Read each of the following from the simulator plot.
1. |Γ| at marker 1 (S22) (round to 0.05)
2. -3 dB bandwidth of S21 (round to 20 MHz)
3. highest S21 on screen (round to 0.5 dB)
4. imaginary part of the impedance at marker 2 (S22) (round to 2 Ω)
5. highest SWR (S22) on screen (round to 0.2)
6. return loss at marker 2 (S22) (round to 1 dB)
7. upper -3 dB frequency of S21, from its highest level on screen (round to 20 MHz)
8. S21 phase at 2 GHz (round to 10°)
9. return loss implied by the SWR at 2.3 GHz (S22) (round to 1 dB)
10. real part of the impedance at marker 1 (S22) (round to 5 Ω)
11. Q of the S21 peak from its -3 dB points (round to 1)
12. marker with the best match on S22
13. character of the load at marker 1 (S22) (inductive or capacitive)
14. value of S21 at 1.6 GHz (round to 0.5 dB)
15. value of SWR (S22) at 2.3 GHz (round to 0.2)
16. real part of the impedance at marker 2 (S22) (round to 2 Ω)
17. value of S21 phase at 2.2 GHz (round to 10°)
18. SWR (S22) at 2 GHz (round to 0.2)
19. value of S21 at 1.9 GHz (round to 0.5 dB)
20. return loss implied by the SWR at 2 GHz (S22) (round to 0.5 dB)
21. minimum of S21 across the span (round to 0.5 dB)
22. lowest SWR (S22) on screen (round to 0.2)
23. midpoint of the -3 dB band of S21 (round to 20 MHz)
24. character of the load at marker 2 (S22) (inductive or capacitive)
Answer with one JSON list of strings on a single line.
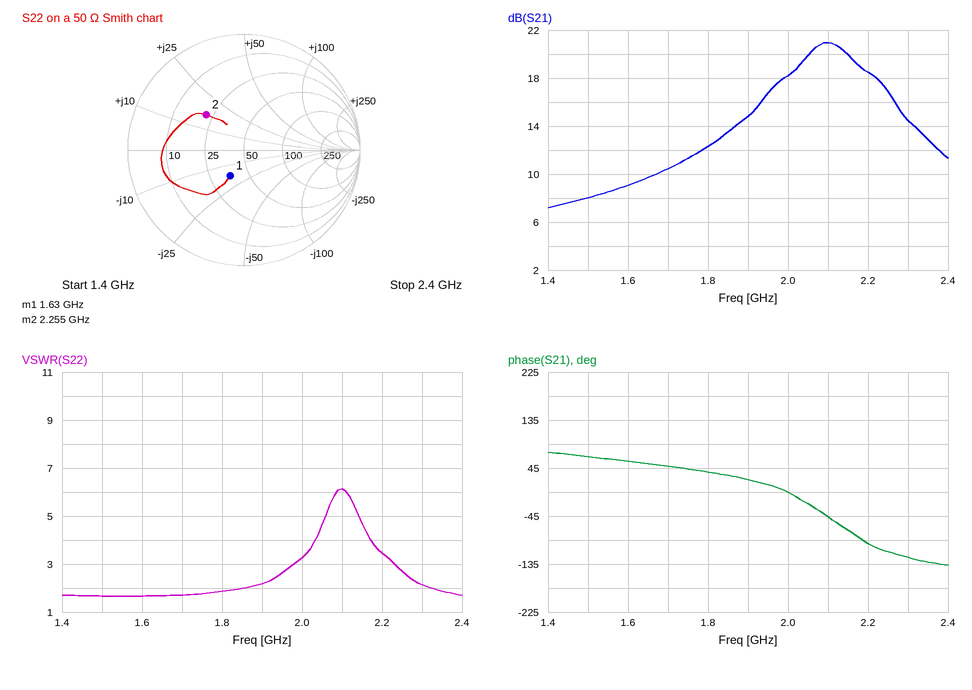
["0.25", "240 MHz", "21.0 dB", "+16 Ω", "6.2", "7 dB", "2.22 GHz", "0°", "9 dB", "35 Ω", "9", "marker 1", "capacitive", "9.0 dB", "2.2", "22 Ω", "-100°", "3.2", "15.0 dB", "5.5 dB", "7.0 dB", "1.6", "2.10 GHz", "inductive"]
